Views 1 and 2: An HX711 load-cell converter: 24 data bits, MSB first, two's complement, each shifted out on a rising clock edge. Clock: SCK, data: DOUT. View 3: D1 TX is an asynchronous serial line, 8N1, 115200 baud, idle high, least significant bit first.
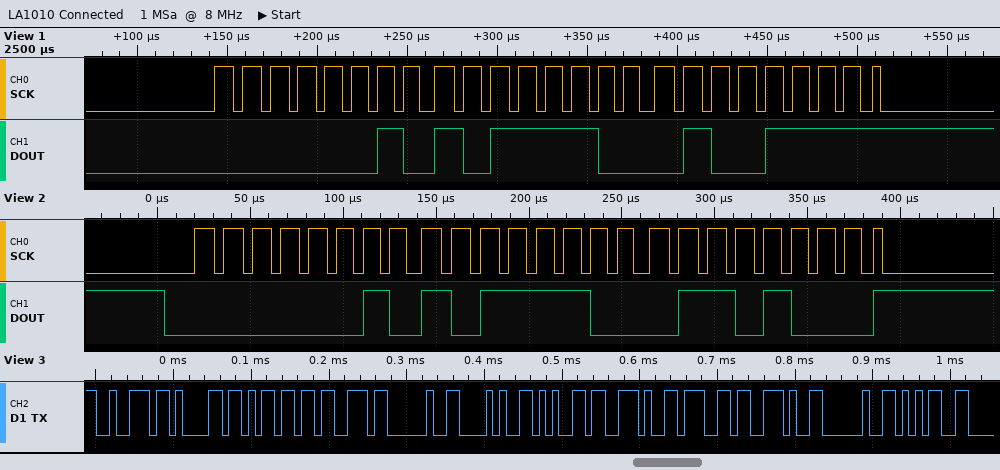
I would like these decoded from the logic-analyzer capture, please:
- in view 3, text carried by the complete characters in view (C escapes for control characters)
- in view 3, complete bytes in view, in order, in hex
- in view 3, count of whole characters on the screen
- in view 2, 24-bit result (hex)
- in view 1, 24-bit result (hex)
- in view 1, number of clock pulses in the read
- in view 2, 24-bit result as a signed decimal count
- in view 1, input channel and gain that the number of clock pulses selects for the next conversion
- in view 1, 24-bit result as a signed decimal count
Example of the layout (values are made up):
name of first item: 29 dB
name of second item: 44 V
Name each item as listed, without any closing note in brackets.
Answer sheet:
in view 3, text carried by the complete characters in view: "rams (e.g. 5"
in view 3, complete bytes in view, in order, in hex: 72 61 6D 73 20 28 65 2E 67 2E 20 35
in view 3, count of whole characters on the screen: 12
in view 2, 24-bit result: 0x02BC68
in view 1, 24-bit result: 0x02BC4F
in view 1, number of clock pulses in the read: 25
in view 2, 24-bit result as a signed decimal count: 179304
in view 1, input channel and gain that the number of clock pulses selects for the next conversion: channel A, gain 128
in view 1, 24-bit result as a signed decimal count: 179279
